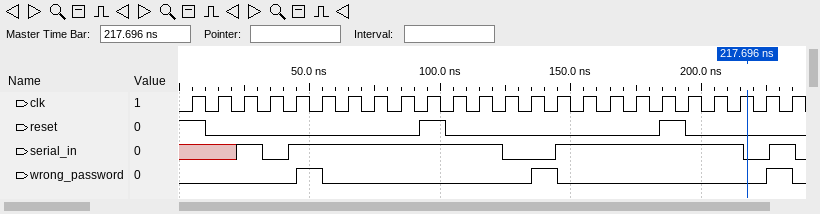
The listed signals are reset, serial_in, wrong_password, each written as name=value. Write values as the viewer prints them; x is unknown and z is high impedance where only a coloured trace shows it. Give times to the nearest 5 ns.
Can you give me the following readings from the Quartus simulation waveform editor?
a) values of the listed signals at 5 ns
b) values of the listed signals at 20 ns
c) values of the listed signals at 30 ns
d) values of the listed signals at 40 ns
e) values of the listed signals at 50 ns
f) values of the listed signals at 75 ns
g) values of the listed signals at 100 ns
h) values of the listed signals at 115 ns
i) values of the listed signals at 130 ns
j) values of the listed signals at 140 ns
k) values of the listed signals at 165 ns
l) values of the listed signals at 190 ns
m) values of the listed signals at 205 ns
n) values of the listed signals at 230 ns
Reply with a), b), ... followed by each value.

a) reset=1, serial_in=x, wrong_password=0
b) reset=0, serial_in=x, wrong_password=0
c) reset=0, serial_in=1, wrong_password=0
d) reset=0, serial_in=0, wrong_password=0
e) reset=0, serial_in=1, wrong_password=1
f) reset=0, serial_in=1, wrong_password=0
g) reset=1, serial_in=1, wrong_password=0
h) reset=0, serial_in=1, wrong_password=0
i) reset=0, serial_in=0, wrong_password=0
j) reset=0, serial_in=0, wrong_password=1
k) reset=0, serial_in=1, wrong_password=0
l) reset=1, serial_in=1, wrong_password=0
m) reset=0, serial_in=1, wrong_password=0
n) reset=0, serial_in=1, wrong_password=1
